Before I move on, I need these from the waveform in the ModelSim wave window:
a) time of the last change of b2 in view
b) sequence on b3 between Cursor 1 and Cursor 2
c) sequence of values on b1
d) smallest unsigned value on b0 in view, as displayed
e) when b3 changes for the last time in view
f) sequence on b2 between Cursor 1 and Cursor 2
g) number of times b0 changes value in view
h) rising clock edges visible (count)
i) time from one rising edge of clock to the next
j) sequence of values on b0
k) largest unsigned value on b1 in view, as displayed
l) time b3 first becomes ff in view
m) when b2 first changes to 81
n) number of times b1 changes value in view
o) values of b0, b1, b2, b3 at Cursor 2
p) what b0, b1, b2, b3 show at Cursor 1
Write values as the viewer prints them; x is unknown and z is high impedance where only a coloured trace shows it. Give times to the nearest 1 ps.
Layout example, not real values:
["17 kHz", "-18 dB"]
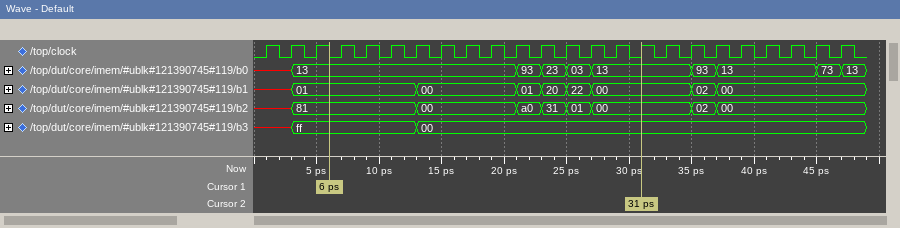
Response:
["37 ps", "ff, 00", "x, 01, 00, 01, 20, 22, 00, 02, 00", "03", "13 ps", "81, 00, a0, 31, 01, 00", "9", "24", "2 ps", "x, 13, 93, 23, 03, 13, 93, 13, 73, 13", "22", "3 ps", "3 ps", "8", "b0=13, b1=00, b2=00, b3=00", "b0=13, b1=01, b2=81, b3=ff"]
